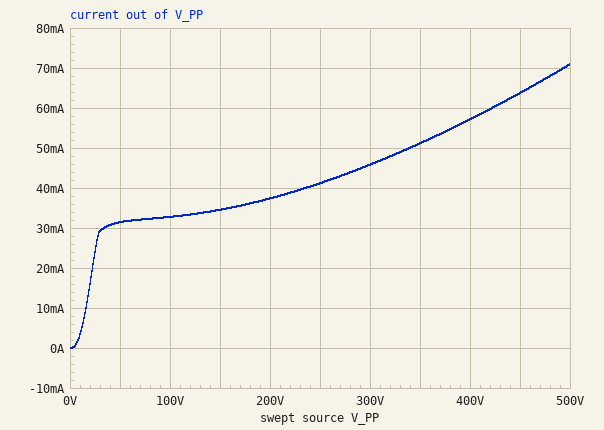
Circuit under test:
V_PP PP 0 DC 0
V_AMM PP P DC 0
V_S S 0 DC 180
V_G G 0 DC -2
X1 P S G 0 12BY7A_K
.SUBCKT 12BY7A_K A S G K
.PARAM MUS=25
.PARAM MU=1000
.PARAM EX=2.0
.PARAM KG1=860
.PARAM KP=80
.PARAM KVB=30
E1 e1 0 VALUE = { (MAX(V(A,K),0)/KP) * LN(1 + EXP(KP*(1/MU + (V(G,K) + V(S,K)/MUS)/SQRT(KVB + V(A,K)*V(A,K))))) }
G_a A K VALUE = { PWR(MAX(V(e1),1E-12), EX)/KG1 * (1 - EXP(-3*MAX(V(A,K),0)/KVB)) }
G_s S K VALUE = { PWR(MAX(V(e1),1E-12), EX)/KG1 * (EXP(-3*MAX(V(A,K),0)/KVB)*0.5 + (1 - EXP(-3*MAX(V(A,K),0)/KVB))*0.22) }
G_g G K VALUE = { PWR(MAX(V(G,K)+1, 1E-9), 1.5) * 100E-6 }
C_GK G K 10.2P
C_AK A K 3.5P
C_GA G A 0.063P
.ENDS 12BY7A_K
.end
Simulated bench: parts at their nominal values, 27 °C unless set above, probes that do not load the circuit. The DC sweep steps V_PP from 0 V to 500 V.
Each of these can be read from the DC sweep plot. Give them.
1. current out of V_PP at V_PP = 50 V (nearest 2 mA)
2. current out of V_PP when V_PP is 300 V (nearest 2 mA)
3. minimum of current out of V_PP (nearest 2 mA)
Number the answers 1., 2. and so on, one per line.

1. 32 mA
2. 46 mA
3. 0 A
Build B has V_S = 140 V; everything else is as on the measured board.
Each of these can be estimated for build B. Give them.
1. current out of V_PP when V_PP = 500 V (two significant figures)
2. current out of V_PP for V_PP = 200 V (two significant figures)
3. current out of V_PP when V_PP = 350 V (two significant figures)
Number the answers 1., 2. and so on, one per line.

1. 52 mA
2. 21 mA
3. 34 mA
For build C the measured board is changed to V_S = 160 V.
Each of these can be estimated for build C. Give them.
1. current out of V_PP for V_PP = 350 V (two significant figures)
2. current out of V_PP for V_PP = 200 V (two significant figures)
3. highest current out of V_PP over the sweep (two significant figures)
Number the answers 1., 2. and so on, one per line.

1. 42 mA
2. 29 mA
3. 61 mA
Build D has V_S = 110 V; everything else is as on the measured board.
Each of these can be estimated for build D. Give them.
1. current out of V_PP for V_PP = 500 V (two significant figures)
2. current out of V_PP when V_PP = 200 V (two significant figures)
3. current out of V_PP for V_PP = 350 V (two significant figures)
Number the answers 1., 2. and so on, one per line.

1. 41 mA
2. 13 mA
3. 25 mA
